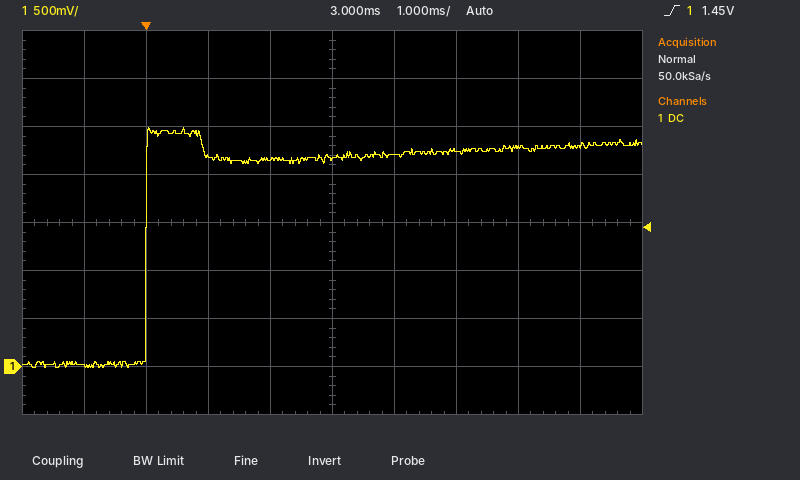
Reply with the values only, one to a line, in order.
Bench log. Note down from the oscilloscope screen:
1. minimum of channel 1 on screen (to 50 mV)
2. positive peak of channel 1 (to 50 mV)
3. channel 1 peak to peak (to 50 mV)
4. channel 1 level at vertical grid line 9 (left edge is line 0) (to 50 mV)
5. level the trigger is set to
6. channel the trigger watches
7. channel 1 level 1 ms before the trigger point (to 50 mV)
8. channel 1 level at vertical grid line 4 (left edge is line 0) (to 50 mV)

0 mV
2.50 V
2.50 V
2.30 V
1.45 V
channel 1
0 mV
2.15 V
